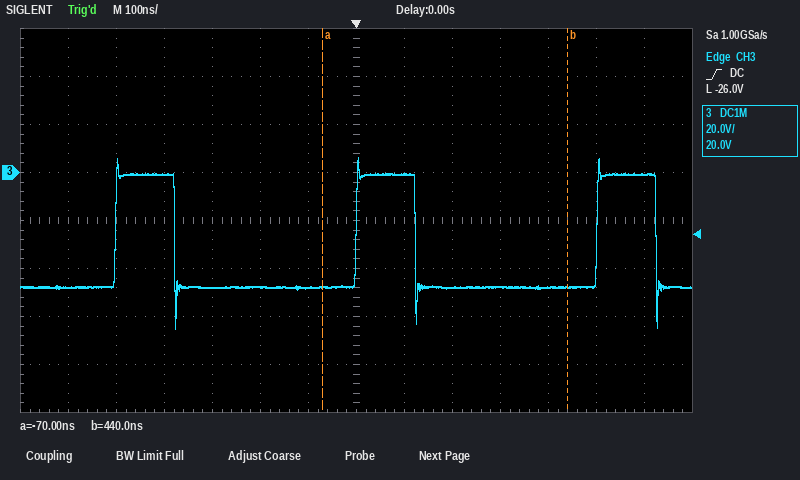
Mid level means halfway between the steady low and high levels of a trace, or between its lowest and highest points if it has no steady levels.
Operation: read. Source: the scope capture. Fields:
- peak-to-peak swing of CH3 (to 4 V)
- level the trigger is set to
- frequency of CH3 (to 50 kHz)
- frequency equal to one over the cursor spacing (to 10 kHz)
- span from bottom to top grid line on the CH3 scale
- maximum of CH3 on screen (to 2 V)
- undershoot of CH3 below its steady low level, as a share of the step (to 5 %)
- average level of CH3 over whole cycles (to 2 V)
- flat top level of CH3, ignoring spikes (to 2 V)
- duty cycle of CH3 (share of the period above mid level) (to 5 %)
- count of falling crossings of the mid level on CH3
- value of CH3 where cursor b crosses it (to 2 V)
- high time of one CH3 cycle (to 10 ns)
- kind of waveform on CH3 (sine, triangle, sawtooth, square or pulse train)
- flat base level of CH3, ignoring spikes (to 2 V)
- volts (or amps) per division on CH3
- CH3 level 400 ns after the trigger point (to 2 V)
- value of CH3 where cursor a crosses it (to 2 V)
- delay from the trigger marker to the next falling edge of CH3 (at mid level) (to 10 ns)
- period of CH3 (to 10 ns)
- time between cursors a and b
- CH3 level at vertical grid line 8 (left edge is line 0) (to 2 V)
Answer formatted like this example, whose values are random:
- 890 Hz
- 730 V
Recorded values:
- 72 V
- -26.0 V
- 2.00 MHz
- 1.96 MHz
- 160 V
- 6 V
- 35 %
- -36 V
- 0 V
- 25 %
- 3
- -48 V
- 120 ns
- pulse train
- -48 V
- 20 V
- -48 V
- -48 V
- 120 ns
- 500 ns
- 510 ns
- 0 V
